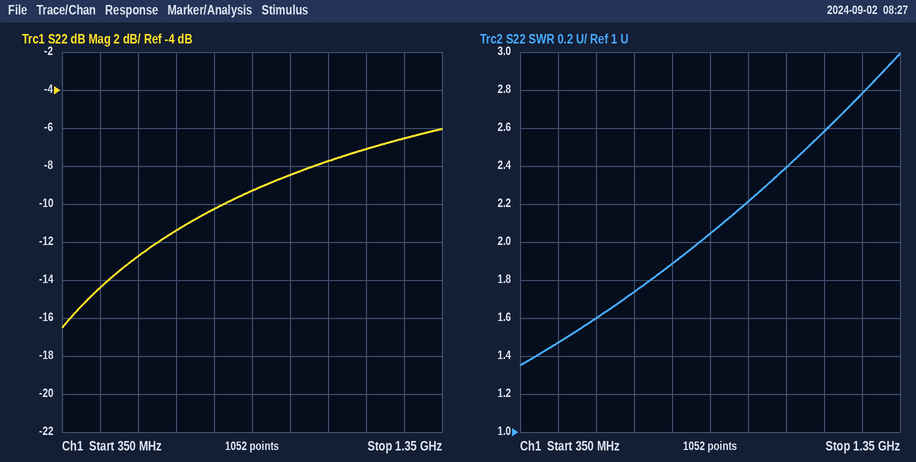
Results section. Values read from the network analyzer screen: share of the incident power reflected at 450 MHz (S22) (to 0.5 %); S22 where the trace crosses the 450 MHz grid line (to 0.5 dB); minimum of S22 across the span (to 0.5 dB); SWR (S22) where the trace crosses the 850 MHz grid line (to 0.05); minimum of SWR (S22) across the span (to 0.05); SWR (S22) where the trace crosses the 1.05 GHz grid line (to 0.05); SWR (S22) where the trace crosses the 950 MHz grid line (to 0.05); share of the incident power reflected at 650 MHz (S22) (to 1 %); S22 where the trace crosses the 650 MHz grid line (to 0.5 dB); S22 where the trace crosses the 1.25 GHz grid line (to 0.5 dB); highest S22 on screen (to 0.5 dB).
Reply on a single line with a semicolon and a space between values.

3.5 %; -14.5 dB; -16.5 dB; 2.05; 1.35; 2.40; 2.20; 7 %; -11.5 dB; -6.5 dB; -6.0 dB
